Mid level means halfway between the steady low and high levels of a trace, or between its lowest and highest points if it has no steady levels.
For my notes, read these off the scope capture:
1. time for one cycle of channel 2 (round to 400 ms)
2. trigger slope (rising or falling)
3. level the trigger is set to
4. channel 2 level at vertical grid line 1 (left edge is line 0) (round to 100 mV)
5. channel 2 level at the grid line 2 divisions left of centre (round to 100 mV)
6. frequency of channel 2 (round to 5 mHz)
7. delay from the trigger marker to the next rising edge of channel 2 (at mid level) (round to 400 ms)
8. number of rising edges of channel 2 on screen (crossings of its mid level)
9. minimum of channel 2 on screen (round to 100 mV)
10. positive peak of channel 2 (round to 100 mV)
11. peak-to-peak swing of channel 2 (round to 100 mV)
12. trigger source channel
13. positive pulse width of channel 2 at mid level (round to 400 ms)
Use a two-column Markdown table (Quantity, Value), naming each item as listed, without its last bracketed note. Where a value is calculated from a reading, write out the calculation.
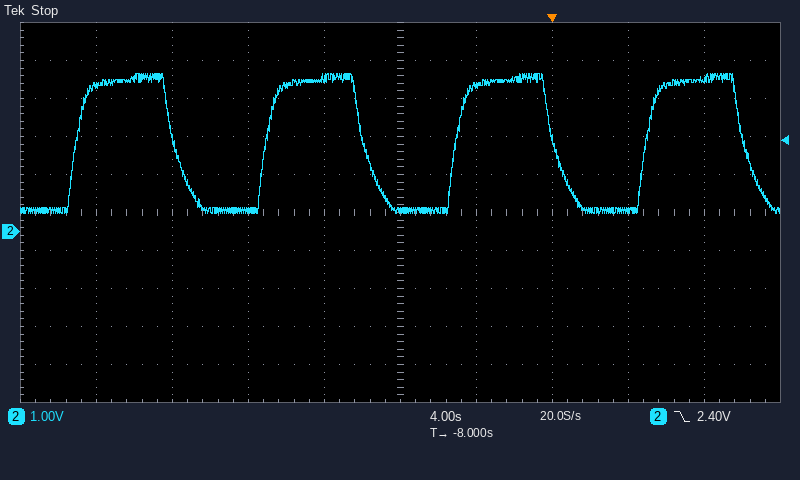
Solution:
| Quantity | Value |
|---|---|
| time for one cycle of channel 2 | 10.0 s |
| trigger slope | falling |
| level the trigger is set to | 2.40 V |
| channel 2 level at vertical grid line 1 (left edge is line 0) | 3.8 V |
| channel 2 level at the grid line 2 divisions left of centre | 600 mV |
| frequency of channel 2 | 1 / 10.0 s ≈ 100 mHz |
| delay from the trigger marker to the next rising edge of channel 2 (at mid level) | 4.8 s |
| number of rising edges of channel 2 on screen | 4 |
| minimum of channel 2 on screen | 500 mV |
| positive peak of channel 2 | 4.2 V |
| peak-to-peak swing of channel 2 | 4.2 V − (500 mV) = 3.7 V |
| trigger source channel | channel 2 |
| positive pulse width of channel 2 at mid level | 5.2 s |
